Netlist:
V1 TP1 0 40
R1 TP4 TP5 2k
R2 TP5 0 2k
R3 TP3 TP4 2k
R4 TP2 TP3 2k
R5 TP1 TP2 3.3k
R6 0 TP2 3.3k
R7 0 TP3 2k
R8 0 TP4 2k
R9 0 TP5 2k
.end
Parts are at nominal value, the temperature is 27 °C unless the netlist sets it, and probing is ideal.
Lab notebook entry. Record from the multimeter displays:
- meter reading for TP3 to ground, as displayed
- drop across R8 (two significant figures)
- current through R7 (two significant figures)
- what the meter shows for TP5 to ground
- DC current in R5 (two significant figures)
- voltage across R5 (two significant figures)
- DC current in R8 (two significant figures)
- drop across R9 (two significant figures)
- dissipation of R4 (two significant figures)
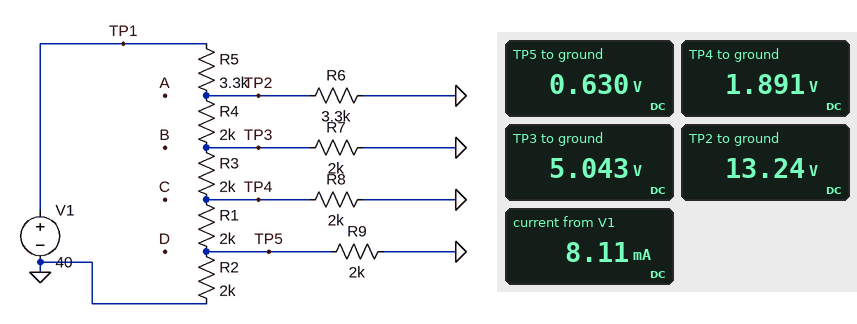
5.043 V
1.9 V
2.5 mA
0.630 V
8.1 mA
27 V
950 µA
630 mV
34 mW
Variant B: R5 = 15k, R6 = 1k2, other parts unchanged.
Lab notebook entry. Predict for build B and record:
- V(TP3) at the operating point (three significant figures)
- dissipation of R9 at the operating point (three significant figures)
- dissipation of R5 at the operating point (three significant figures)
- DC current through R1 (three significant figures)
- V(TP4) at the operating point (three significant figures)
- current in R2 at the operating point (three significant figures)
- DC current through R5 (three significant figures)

840 mV
5.51 µW
95.2 mW
105 µA
315 mV
52.5 µA
2.52 mA
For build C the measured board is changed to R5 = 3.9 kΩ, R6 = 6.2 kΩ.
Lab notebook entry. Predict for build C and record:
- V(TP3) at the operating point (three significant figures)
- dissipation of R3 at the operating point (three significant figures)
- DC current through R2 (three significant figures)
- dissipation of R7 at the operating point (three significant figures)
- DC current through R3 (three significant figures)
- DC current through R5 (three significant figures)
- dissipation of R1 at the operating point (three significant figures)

5.37 V
5.64 mW
336 µA
14.4 mW
1.68 mA
6.64 mA
902 µW
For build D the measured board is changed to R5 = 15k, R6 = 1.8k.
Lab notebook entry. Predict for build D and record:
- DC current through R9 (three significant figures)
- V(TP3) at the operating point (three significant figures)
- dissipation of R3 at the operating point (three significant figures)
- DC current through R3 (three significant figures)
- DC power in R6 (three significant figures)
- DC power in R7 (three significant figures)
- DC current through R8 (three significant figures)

68.1 µA
1.09 V
232 µW
341 µA
4.55 mW
594 µW
204 µA
